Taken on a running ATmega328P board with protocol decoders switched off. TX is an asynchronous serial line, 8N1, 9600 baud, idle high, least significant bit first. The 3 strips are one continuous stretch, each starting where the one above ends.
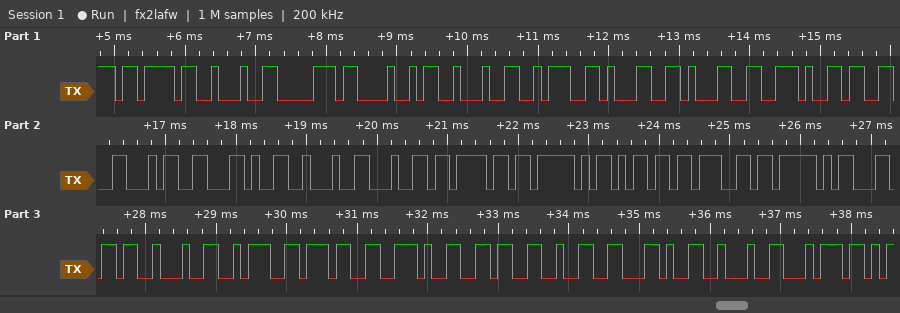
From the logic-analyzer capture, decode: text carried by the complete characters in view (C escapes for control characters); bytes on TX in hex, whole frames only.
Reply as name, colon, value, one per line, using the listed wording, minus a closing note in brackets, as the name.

text carried by the complete characters in view: "{\"pH\":11.34,\"do_mg_l\":7.62,\"t"
bytes on TX in hex, whole frames only: 7B 22 70 48 22 3A 31 31 2E 33 34 2C 22 64 6F 5F 6D 67 5F 6C 22 3A 37 2E 36 32 2C 22 74
